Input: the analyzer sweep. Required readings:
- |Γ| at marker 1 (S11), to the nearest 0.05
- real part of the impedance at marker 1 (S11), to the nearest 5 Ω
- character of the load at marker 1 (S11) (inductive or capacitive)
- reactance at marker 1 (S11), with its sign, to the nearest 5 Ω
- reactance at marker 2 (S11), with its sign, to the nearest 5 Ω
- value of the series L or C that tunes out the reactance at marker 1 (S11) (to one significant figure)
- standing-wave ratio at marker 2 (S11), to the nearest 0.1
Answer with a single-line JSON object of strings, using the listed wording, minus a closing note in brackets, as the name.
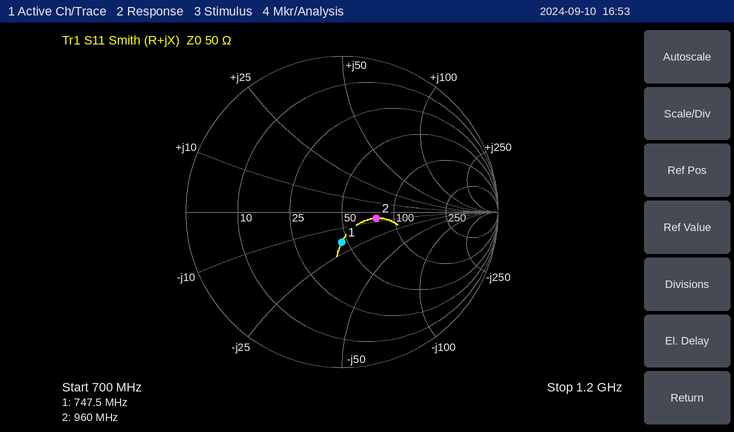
{"|Γ| at marker 1 (S11), to the nearest 0.05": "0.20", "real part of the impedance at marker 1 (S11), to the nearest 5 Ω": "45 Ω", "character of the load at marker 1 (S11)": "capacitive", "reactance at marker 1 (S11), with its sign, to the nearest 5 Ω": "-20 Ω", "reactance at marker 2 (S11), with its sign, to the nearest 5 Ω": "-5 Ω", "value of the series L or C that tunes out the reactance at marker 1 (S11)": "4 nH", "standing-wave ratio at marker 2 (S11), to the nearest 0.1": "1.6"}
